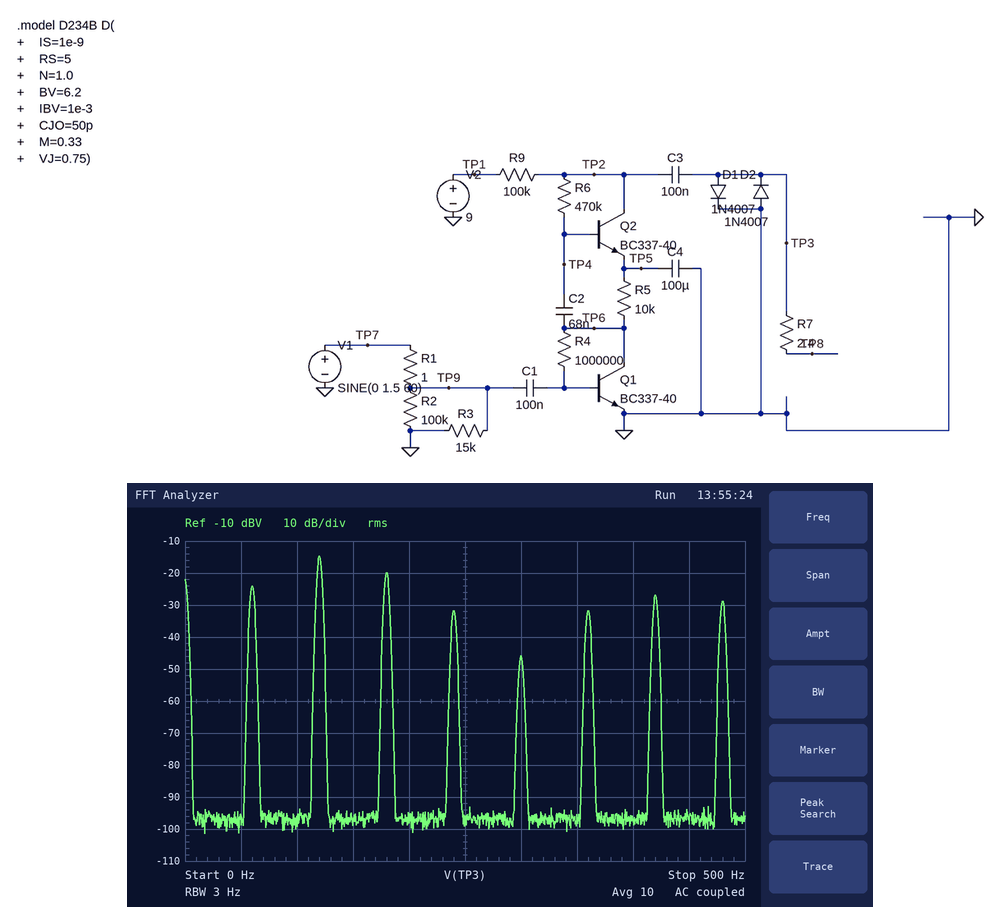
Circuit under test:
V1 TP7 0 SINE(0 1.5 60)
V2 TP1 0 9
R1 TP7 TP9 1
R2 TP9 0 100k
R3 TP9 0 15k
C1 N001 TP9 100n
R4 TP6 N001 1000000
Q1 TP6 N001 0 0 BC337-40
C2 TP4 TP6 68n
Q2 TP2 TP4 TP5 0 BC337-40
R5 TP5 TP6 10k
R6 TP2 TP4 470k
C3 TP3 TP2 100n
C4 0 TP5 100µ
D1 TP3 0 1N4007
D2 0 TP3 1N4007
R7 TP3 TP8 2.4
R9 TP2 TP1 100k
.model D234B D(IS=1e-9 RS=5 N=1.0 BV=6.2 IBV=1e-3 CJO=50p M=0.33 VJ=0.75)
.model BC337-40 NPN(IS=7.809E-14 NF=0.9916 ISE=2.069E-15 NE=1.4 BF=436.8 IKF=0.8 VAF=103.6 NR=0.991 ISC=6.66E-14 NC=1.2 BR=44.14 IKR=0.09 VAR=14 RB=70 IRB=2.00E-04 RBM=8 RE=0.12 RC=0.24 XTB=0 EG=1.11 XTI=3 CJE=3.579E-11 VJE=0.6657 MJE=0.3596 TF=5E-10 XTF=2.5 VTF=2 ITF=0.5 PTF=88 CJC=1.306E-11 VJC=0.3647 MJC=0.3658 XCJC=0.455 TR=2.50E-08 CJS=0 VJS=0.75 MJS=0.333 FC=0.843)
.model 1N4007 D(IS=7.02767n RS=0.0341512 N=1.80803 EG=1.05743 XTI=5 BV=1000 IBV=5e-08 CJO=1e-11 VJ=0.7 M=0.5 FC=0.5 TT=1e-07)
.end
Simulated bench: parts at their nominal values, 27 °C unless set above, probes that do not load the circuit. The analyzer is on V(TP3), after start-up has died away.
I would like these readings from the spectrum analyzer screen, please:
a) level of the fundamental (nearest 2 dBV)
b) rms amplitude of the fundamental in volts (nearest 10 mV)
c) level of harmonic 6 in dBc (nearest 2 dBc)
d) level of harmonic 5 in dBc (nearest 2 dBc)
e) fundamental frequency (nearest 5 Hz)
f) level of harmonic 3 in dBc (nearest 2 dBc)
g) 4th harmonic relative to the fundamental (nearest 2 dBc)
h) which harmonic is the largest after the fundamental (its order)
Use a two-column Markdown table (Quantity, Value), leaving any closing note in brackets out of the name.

| Quantity | Value |
|---|---|
| level of the fundamental | -24 dBV |
| rms amplitude of the fundamental in volts | 60 mV |
| level of harmonic 6 in dBc | -8 dBc |
| level of harmonic 5 in dBc | -22 dBc |
| fundamental frequency | 60 Hz |
| level of harmonic 3 in dBc | 4 dBc |
| 4th harmonic relative to the fundamental | -8 dBc |
| which harmonic is the largest after the fundamental | 2 |
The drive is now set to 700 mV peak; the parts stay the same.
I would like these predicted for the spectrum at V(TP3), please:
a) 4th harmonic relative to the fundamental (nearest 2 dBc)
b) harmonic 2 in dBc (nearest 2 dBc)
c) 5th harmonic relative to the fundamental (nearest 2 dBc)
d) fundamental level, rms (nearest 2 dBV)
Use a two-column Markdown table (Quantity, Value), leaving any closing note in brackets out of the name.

| Quantity | Value |
|---|---|
| 4th harmonic relative to the fundamental | -20 dBc |
| harmonic 2 in dBc | 2 dBc |
| 5th harmonic relative to the fundamental | -12 dBc |
| fundamental level, rms | -18 dBV |
